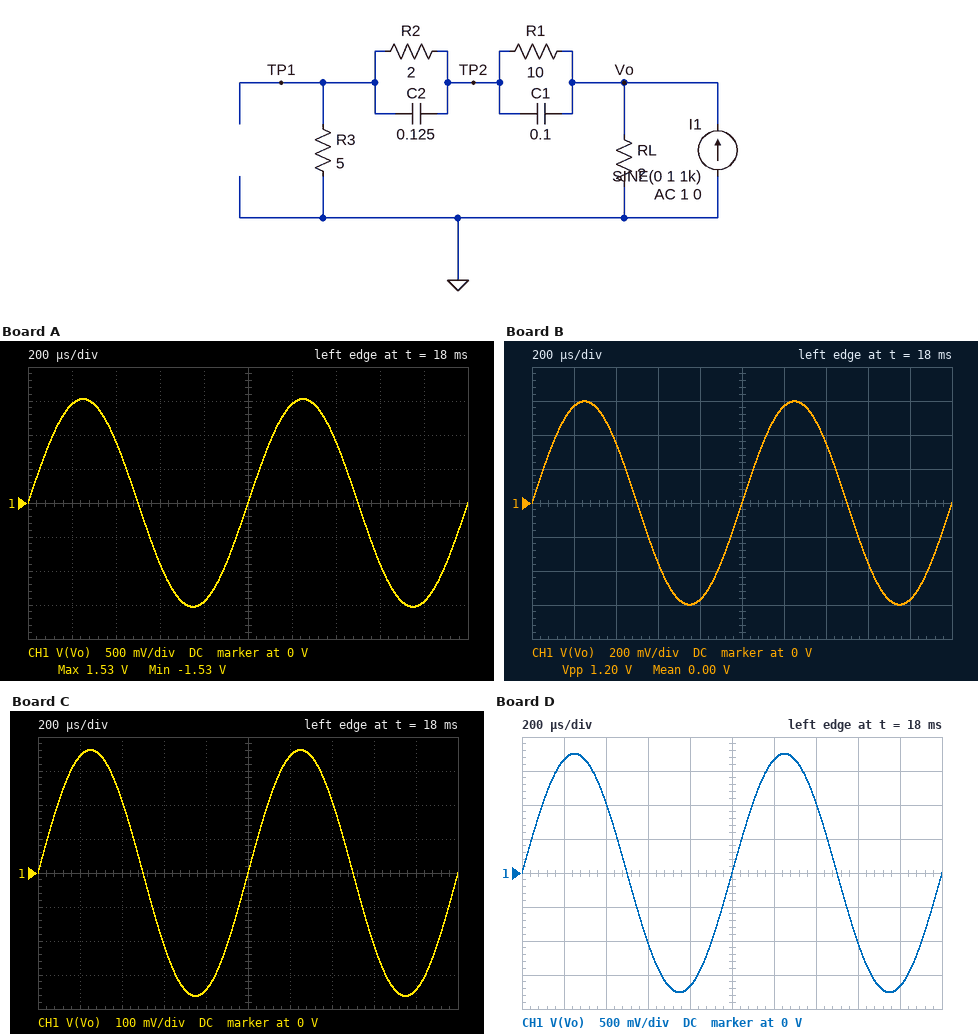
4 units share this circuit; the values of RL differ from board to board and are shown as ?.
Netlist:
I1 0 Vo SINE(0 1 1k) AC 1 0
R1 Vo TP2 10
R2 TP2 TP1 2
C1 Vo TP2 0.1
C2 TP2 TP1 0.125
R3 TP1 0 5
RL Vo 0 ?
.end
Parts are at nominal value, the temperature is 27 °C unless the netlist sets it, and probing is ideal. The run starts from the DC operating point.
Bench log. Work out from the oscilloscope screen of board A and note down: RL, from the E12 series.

2.2 Ω
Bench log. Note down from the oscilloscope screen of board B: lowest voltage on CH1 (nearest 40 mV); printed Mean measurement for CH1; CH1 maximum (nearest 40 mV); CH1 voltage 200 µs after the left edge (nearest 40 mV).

-600 mV
0.00 V
600 mV
560 mV
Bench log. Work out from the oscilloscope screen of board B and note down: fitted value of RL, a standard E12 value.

0.68 Ω
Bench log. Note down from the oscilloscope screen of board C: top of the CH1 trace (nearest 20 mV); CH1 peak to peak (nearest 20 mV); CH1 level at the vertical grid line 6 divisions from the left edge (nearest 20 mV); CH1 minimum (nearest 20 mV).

360 mV
720 mV
340 mV
-360 mV
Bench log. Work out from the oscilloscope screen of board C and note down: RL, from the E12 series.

0.39 Ω
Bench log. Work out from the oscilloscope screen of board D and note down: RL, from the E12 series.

2.7 Ω
